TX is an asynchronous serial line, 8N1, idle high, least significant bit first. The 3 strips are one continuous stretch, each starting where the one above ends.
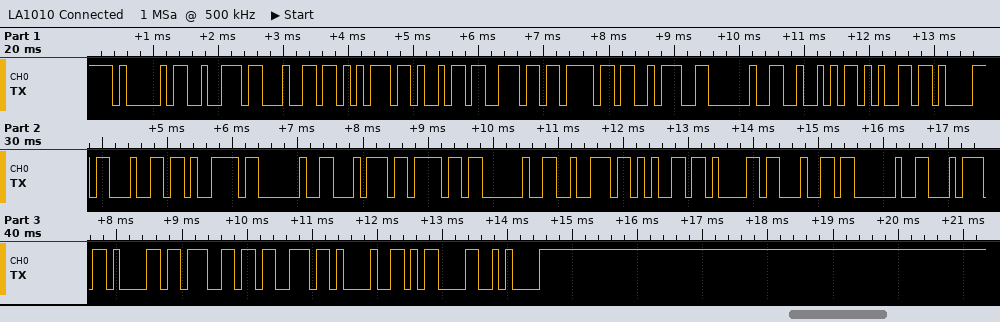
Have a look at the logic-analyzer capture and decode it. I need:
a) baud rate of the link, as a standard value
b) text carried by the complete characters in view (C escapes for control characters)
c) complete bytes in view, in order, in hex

9600 baud
"Arduino: Ready to read tags!\r\n"
41 72 64 75 69 6E 6F 3A 20 52 65 61 64 79 20 74 6F 20 72 65 61 64 20 74 61 67 73 21 0D 0A
